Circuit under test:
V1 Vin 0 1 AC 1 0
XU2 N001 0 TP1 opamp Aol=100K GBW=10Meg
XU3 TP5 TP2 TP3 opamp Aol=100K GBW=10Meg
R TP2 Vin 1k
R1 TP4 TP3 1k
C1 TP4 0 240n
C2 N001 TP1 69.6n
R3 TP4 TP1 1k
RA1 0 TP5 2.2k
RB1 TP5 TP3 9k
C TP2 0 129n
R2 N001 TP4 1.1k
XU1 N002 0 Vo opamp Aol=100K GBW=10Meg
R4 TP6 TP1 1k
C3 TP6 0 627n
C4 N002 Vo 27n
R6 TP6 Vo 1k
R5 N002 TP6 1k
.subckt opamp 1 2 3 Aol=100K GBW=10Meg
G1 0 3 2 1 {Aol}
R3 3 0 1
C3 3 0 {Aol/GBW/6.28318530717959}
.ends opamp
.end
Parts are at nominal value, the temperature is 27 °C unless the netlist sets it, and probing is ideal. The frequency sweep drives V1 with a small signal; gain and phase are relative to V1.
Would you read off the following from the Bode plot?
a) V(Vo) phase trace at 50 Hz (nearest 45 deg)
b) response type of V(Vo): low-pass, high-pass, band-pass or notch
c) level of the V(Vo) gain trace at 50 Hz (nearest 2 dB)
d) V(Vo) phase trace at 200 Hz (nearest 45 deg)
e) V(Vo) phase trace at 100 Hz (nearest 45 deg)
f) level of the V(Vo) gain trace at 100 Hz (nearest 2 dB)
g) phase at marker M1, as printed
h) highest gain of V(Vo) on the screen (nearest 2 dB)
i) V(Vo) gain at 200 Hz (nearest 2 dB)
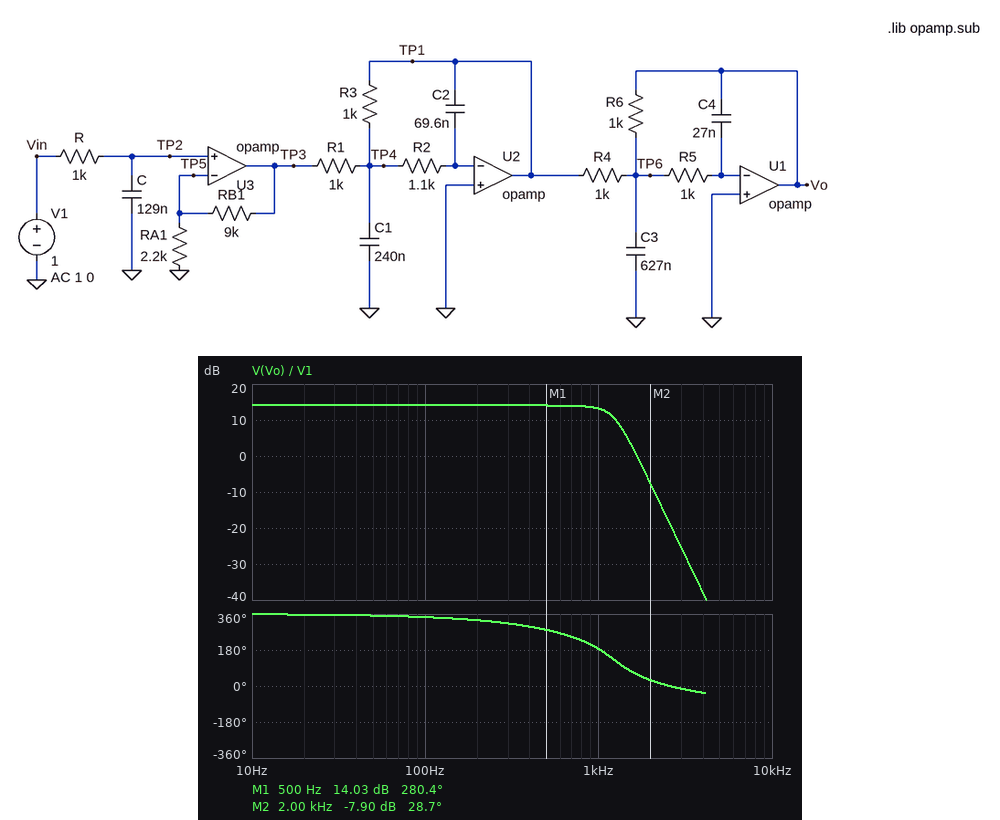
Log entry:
360 deg
low-pass
14 dB
315 deg
360 deg
14 dB
280.4 deg
14 dB
14 dB
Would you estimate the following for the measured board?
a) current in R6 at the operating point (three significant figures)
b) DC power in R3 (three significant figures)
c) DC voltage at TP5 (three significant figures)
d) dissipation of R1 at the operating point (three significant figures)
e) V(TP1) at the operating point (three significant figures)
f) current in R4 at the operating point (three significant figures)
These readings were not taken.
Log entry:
5.09 mA
25.9 mW
1.00 V
25.9 mW
-5.09 V
5.09 mA
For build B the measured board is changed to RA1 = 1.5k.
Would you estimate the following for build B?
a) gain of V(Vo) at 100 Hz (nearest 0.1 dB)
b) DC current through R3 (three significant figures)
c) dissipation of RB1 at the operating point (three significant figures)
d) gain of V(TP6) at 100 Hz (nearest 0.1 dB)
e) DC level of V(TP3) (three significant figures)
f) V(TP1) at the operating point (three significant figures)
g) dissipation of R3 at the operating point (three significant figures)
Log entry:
16.9 dB
7.00 mA
4.00 mW
-18.5 dB
7.00 V
-7.00 V
49.0 mW
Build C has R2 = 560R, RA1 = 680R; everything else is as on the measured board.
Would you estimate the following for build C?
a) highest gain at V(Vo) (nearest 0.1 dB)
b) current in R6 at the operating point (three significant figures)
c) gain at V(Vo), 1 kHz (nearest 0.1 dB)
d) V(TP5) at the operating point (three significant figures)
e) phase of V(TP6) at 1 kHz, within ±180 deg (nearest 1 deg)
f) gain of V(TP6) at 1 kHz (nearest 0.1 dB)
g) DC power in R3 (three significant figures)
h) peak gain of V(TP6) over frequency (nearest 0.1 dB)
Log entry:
24.3 dB
14.2 mA
24.2 dB
1.00 V
118 deg
8.8 dB
203 mW
9.2 dB
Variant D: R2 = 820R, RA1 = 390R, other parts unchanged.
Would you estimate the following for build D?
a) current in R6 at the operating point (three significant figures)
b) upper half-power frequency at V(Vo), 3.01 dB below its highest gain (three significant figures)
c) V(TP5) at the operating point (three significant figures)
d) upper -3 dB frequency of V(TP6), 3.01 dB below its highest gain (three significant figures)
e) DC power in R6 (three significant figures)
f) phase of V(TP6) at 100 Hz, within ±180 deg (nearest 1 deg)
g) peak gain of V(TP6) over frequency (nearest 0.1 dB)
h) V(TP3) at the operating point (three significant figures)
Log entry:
24.1 mA
1.26 kHz
1.00 V
1.39 kHz
579 mW
-104 deg
12.7 dB
24.1 V
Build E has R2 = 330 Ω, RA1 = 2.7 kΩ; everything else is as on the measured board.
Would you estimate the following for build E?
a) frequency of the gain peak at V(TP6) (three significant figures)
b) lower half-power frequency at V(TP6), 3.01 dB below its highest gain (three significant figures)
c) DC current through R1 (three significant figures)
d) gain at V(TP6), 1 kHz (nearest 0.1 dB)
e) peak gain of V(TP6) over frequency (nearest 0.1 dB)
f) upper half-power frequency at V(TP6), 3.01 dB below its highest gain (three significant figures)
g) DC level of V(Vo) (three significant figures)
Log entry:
1.14 kHz
792 Hz
4.33 mA
-1.1 dB
-0.5 dB
1.47 kHz
4.33 V
